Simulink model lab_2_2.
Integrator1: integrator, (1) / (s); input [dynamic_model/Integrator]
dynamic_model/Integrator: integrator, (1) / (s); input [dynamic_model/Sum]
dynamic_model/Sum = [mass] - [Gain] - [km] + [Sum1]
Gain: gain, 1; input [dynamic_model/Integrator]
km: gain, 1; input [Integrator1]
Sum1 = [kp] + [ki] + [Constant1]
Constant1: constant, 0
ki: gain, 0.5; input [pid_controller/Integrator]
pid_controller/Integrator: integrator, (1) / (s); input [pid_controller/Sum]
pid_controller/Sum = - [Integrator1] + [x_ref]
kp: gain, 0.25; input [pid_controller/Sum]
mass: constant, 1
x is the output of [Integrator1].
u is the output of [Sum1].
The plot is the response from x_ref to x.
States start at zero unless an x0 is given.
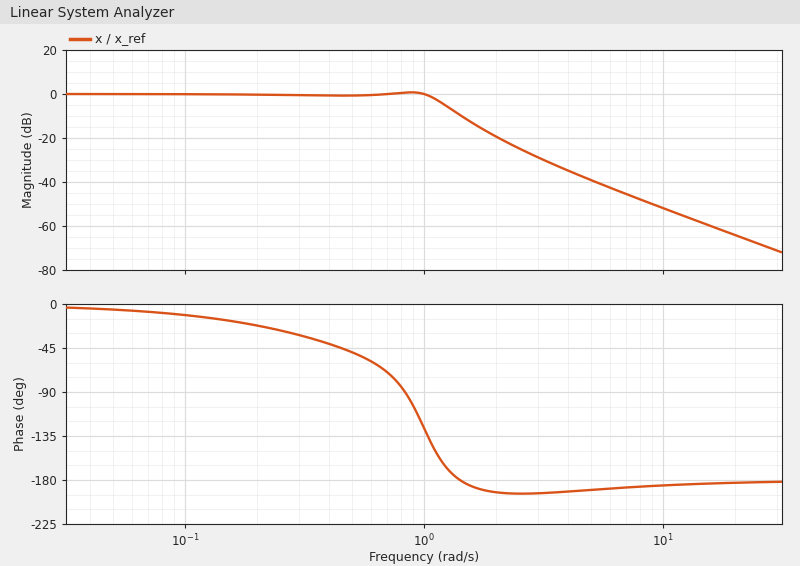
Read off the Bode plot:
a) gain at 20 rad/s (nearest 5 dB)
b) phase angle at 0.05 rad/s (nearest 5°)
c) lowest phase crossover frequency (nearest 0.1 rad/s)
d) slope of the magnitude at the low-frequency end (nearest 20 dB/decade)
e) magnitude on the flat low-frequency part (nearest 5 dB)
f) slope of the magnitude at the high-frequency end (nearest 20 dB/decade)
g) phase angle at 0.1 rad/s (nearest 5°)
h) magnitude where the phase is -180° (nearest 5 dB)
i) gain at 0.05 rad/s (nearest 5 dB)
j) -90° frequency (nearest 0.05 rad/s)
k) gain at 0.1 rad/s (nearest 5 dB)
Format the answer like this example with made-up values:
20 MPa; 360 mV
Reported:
-65 dB; -5°; 1.4 rad/s; 0 dB/decade; 0 dB; -40 dB/decade; -10°; -10 dB; 0 dB; 0.85 rad/s; 0 dB
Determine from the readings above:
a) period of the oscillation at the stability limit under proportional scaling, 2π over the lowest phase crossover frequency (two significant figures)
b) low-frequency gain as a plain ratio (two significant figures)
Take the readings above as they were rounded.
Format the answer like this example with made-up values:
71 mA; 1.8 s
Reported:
4.5 s; 1.0
